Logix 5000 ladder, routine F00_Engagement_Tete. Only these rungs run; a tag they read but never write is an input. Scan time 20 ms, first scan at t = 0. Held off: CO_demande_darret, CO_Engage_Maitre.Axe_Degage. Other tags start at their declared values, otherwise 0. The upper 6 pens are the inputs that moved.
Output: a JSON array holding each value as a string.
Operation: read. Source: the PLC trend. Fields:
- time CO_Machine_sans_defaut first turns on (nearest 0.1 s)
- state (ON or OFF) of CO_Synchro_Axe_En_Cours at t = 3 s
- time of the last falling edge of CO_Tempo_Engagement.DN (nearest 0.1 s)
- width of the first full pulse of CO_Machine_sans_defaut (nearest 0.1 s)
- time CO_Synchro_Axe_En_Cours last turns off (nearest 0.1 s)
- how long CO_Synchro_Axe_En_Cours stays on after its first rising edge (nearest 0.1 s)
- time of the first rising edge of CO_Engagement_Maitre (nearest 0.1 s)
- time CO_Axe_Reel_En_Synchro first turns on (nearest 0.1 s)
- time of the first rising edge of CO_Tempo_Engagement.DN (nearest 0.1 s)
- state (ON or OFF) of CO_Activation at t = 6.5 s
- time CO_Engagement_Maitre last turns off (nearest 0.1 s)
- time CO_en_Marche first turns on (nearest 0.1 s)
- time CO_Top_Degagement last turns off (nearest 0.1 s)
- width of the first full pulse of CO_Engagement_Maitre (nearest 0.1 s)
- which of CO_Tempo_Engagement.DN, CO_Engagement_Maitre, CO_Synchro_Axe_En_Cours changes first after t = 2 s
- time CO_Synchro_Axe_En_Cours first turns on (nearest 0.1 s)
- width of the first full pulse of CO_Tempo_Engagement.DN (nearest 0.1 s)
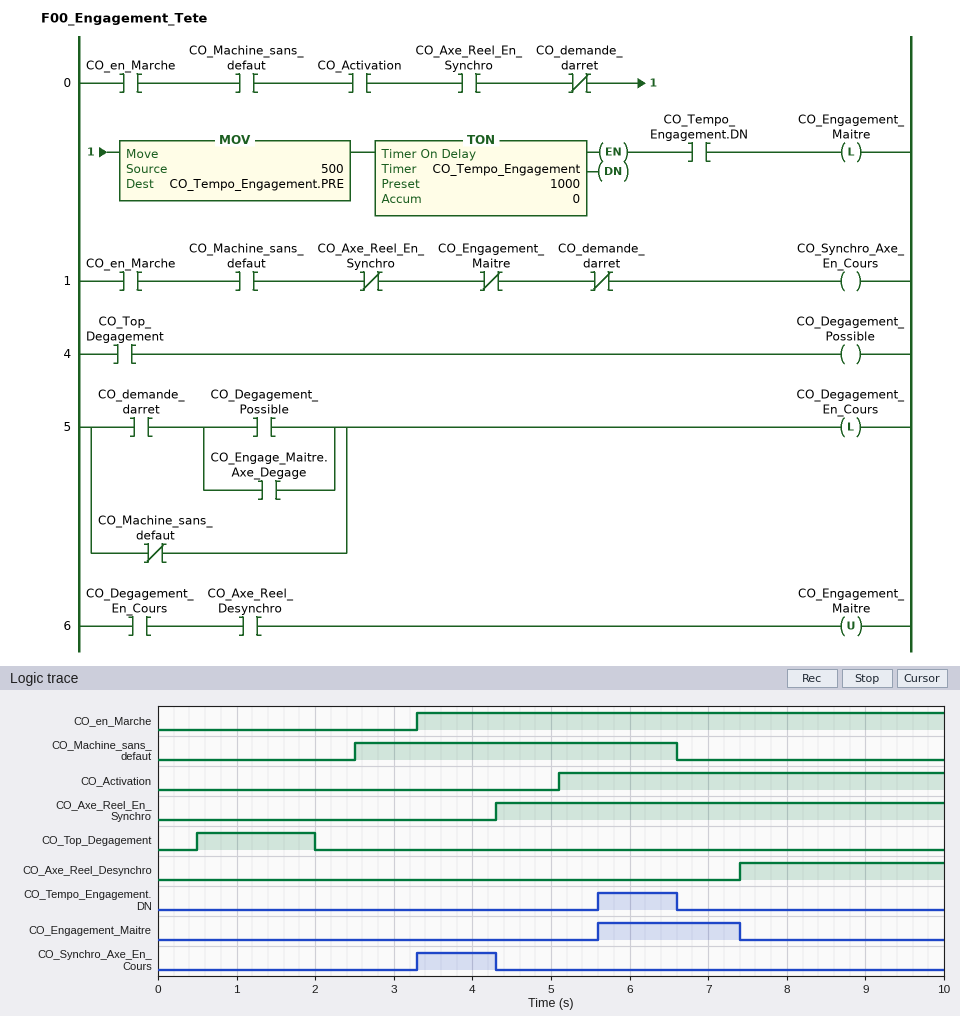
["2.5 s", "OFF", "6.6 s", "4.1 s", "4.3 s", "1.0 s", "5.6 s", "4.3 s", "5.6 s", "ON", "7.4 s", "3.3 s", "2.0 s", "1.8 s", "CO_Synchro_Axe_En_Cours", "3.3 s", "1.0 s"]
